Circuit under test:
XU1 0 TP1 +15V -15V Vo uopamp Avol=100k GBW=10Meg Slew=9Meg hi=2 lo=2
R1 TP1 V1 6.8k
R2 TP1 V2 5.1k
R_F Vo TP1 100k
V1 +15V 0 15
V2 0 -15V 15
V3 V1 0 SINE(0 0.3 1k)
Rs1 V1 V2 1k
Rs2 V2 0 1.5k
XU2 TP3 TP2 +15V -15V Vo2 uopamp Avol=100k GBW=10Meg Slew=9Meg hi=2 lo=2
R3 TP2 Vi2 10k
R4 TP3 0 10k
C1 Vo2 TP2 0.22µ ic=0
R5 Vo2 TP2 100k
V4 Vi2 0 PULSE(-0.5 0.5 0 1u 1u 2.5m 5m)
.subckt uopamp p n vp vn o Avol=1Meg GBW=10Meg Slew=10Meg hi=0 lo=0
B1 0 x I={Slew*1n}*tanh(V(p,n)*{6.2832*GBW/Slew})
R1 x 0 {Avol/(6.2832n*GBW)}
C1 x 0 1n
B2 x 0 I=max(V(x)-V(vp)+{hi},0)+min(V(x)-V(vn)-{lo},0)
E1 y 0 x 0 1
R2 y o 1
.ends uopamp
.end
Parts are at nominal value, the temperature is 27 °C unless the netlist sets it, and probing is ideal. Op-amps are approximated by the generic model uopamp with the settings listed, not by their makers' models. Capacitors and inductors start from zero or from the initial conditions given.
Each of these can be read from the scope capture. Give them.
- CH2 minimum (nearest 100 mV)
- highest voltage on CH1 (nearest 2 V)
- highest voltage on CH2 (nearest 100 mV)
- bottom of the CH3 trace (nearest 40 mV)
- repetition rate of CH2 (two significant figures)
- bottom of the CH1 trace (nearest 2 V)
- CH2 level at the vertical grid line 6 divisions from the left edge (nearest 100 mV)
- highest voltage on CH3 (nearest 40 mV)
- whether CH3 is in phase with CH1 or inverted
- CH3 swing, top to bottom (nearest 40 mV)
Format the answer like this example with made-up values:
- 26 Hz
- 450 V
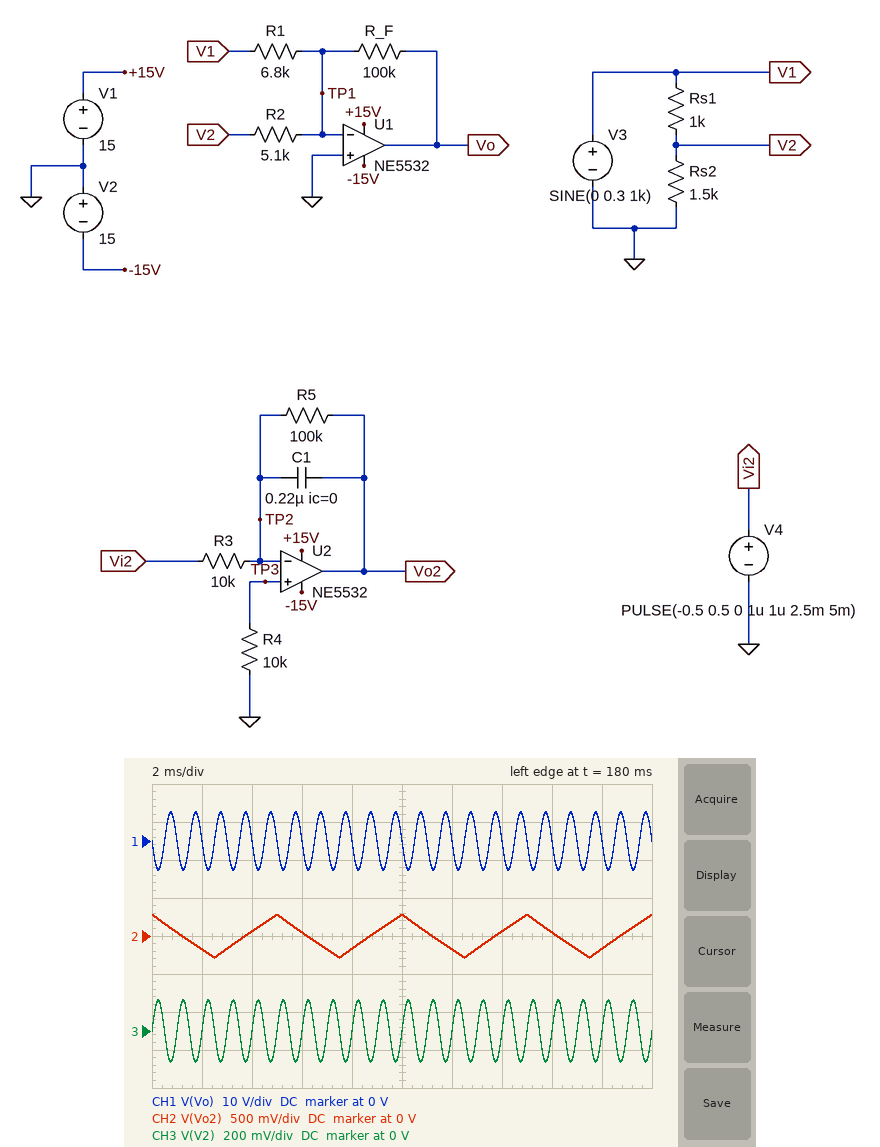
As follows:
- -300 mV
- 8 V
- 300 mV
- -160 mV
- 200 Hz
- -8 V
- -200 mV
- 160 mV
- inverted
- 320 mV
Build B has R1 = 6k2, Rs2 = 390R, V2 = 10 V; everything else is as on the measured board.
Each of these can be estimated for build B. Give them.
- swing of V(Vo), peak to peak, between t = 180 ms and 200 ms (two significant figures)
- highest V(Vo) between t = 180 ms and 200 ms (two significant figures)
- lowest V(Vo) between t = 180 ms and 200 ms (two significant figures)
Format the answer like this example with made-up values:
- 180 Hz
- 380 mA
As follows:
- 13 V
- 6.4 V
- -6.4 V
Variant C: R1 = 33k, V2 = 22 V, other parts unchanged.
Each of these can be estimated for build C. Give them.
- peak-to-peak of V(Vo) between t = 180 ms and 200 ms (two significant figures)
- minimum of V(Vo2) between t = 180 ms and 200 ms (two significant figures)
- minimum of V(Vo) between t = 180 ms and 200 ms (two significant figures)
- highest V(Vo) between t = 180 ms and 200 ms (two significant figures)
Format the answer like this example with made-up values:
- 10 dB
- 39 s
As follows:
- 8.1 V
- -290 mV
- -4.1 V
- 4.1 V
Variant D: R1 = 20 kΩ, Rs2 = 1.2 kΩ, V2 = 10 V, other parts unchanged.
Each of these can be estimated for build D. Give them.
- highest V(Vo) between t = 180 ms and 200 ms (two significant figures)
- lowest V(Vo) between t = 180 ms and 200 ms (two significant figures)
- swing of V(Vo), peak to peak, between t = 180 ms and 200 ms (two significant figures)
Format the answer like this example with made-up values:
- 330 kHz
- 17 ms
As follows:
- 4.4 V
- -4.4 V
- 8.8 V
